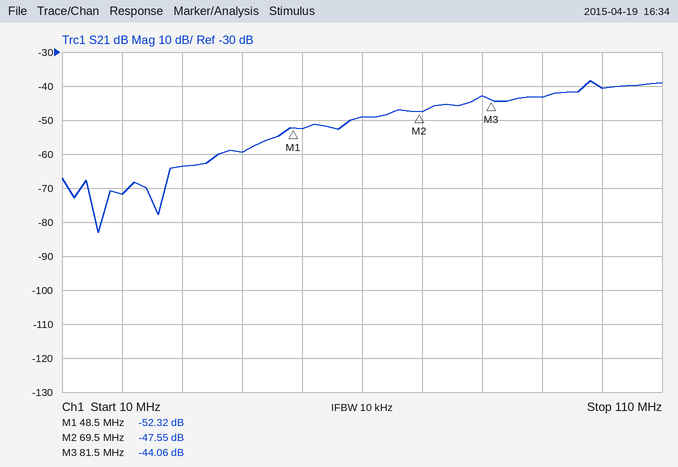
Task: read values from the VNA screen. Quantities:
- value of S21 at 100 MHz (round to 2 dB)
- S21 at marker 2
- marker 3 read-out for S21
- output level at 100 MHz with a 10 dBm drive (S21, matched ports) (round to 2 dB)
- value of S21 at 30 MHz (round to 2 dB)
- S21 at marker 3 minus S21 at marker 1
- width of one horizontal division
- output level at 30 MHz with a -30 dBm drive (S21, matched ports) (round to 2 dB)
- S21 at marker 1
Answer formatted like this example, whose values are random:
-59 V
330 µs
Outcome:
-40 dB
-47.55 dB
-44.06 dB
-30 dBm
-64 dB
8.26 dB
10 MHz
-94 dBm
-52.32 dB
